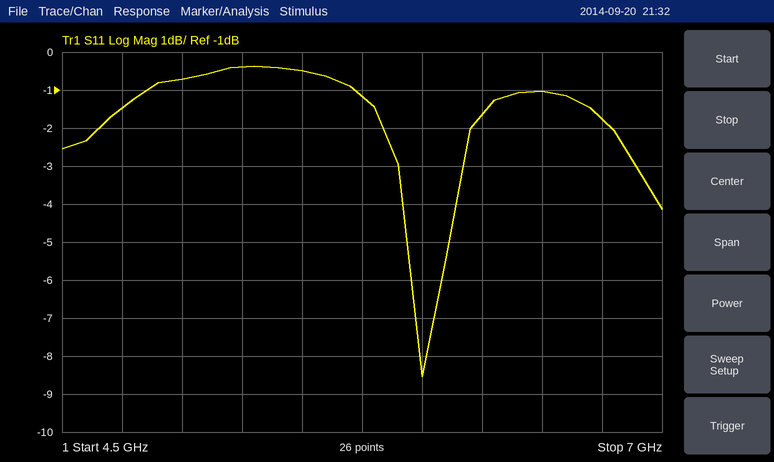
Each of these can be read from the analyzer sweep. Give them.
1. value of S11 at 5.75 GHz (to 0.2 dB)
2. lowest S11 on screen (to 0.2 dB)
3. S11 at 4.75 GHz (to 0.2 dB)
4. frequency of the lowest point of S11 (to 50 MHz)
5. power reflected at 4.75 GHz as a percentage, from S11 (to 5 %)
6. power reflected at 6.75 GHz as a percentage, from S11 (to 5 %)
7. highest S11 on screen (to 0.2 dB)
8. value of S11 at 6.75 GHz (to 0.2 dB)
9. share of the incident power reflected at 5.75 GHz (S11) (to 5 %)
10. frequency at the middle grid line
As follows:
-1.2 dB
-8.6 dB
-1.4 dB
6.00 GHz
70 %
65 %
-0.4 dB
-1.8 dB
75 %
5.75 GHz
